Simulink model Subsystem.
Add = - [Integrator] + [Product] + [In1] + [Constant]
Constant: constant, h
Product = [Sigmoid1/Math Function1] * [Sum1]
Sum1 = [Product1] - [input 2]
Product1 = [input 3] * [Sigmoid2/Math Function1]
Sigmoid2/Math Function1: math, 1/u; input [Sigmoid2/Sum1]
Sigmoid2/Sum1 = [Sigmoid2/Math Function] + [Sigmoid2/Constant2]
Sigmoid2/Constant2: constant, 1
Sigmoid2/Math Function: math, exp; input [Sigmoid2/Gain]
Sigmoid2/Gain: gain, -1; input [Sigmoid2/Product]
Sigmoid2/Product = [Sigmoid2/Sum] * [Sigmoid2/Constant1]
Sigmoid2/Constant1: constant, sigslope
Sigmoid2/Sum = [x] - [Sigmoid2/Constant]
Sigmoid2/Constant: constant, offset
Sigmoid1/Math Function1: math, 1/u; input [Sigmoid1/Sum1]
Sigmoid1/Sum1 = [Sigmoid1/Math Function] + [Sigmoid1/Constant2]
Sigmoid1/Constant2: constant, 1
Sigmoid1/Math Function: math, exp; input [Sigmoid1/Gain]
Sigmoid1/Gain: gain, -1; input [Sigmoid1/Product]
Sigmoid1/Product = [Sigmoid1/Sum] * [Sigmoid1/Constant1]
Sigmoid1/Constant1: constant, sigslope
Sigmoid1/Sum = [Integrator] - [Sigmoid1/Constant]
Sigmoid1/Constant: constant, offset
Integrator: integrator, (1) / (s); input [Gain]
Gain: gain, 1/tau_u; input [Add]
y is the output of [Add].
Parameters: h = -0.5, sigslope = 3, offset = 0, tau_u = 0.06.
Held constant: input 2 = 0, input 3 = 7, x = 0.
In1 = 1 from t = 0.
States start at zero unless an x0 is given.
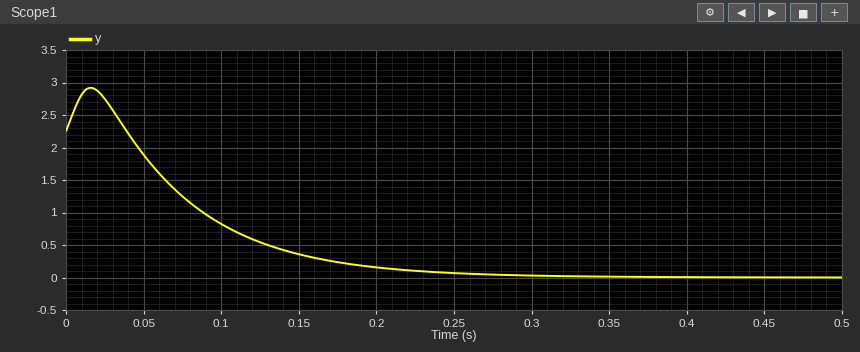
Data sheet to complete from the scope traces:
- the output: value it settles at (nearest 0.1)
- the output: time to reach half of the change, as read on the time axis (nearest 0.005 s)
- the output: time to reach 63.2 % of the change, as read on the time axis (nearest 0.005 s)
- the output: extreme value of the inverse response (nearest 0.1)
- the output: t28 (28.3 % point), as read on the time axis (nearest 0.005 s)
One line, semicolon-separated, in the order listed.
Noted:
0.0; 0.080 s; 0.100 s; 2.9; 0.060 s
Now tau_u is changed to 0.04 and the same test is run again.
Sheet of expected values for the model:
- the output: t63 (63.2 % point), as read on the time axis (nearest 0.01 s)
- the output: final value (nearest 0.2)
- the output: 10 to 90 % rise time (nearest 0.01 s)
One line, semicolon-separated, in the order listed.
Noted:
0.07 s; 0.0; 0.09 s
